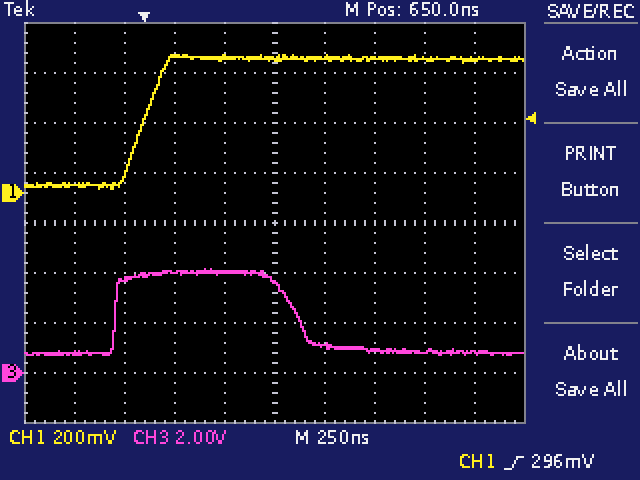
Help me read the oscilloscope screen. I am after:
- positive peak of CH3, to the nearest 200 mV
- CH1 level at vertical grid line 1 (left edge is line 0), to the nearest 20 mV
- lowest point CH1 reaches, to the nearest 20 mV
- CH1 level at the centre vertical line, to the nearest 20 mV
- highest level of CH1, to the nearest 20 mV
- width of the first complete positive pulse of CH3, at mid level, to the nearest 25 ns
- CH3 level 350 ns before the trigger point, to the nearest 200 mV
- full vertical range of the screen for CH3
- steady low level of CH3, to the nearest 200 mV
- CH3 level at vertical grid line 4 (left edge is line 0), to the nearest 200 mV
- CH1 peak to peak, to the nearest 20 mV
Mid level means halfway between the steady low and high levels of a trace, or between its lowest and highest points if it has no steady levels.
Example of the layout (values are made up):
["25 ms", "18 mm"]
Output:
["4.2 V", "40 mV", "20 mV", "540 mV", "560 mV", "900 ns", "800 mV", "16 V", "800 mV", "4.0 V", "540 mV"]
